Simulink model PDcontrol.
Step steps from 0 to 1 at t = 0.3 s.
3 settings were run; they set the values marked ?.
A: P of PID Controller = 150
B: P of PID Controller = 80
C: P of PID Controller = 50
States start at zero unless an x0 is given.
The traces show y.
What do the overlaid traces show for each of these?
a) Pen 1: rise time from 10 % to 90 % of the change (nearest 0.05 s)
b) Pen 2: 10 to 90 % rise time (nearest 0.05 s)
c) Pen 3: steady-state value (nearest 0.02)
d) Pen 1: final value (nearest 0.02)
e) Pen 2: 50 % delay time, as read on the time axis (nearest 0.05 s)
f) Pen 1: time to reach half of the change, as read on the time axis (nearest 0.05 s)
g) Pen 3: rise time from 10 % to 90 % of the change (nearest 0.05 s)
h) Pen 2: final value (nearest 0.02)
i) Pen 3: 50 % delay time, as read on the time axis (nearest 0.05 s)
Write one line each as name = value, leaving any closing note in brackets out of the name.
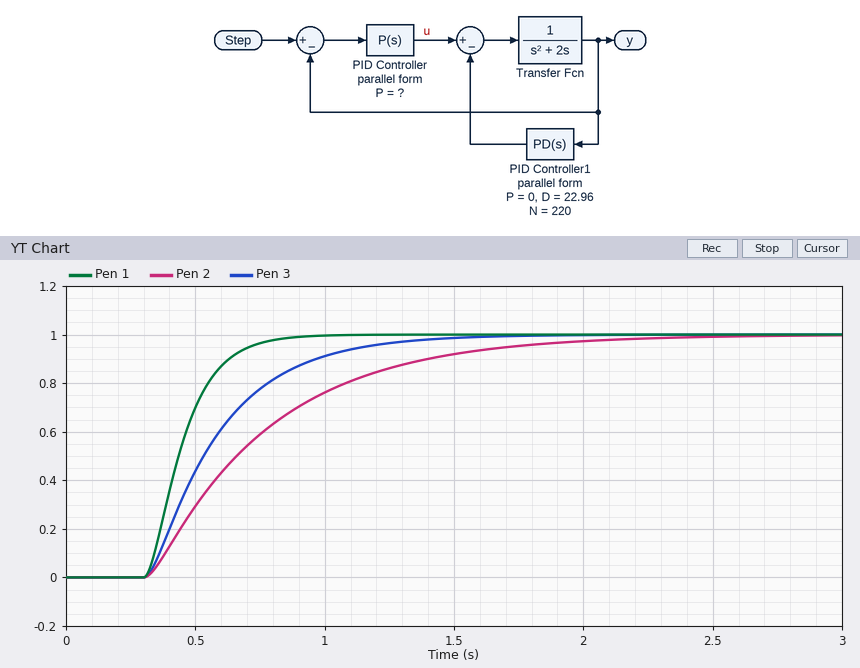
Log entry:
Pen 1: rise time from 10 % to 90 % of the change = 0.30 s
Pen 2: 10 to 90 % rise time = 1.00 s
Pen 3: steady-state value = 1.00
Pen 1: final value = 1.00
Pen 2: 50 % delay time, as read on the time axis = 0.65 s
Pen 1: time to reach half of the change, as read on the time axis = 0.45 s
Pen 3: rise time from 10 % to 90 % of the change = 0.60 s
Pen 2: final value = 1.00
Pen 3: 50 % delay time, as read on the time axis = 0.55 s
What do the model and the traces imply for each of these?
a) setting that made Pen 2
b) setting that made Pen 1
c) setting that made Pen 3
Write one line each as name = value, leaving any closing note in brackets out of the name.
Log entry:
setting that made Pen 2 = C
setting that made Pen 1 = A
setting that made Pen 3 = B
